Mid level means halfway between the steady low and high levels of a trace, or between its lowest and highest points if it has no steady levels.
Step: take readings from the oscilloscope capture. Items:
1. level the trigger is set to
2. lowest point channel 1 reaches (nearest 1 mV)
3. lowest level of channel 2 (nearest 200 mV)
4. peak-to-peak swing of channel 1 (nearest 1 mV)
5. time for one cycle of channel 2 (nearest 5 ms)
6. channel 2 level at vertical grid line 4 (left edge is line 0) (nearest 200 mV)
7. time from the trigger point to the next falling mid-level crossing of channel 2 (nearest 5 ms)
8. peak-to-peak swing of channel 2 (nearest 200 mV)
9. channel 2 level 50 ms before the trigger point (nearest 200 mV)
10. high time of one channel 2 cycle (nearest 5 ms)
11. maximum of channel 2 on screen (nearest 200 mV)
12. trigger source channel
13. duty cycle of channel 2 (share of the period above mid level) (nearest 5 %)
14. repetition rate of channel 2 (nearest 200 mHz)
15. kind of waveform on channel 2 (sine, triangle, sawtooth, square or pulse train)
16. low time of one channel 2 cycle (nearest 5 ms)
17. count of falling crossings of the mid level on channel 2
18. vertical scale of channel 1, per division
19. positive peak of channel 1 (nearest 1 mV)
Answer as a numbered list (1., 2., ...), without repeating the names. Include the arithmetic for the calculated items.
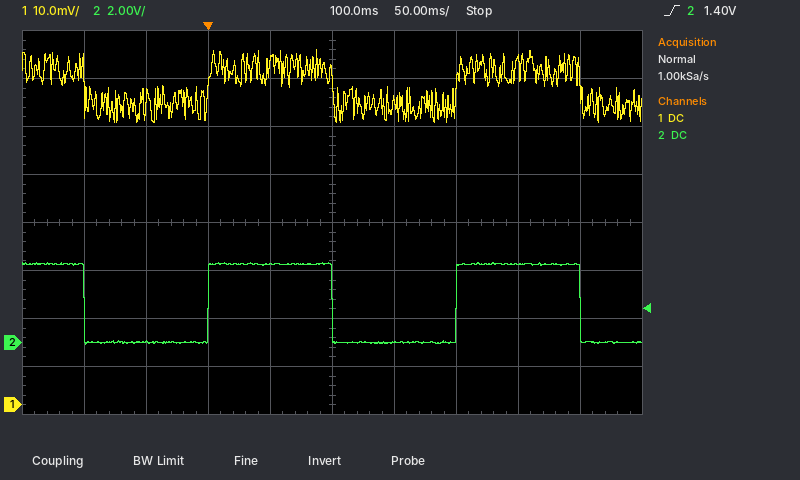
1. 1.40 V
2. 59 mV
3. 0.0 V
4. 74 mV − (59 mV) = 15 mV
5. 200 ms
6. 3.2 V
7. 100 ms
8. 3.4 V − (0.0 V) = 3.4 V
9. 0.0 V
10. 100 ms
11. 3.4 V
12. channel 2
13. 100 ms / 200 ms ≈ 50 %
14. 1 / 200 ms ≈ 5.0 Hz
15. square
16. 100 ms
17. 3
18. 10 mV
19. 74 mV
